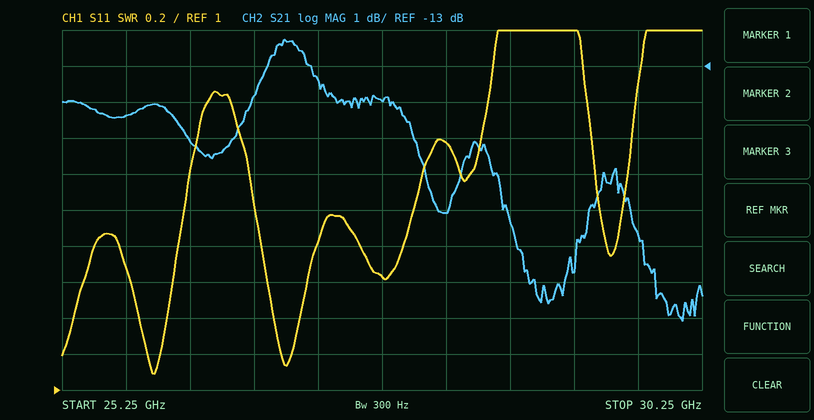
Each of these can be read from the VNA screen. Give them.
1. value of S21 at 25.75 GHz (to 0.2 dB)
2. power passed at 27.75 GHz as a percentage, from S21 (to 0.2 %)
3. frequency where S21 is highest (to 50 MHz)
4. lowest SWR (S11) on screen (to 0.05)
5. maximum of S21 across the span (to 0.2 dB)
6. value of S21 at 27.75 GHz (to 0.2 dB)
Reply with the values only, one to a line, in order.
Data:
-14.4 dB
4.0 %
27.00 GHz
1.10
-12.2 dB
-14.0 dB
